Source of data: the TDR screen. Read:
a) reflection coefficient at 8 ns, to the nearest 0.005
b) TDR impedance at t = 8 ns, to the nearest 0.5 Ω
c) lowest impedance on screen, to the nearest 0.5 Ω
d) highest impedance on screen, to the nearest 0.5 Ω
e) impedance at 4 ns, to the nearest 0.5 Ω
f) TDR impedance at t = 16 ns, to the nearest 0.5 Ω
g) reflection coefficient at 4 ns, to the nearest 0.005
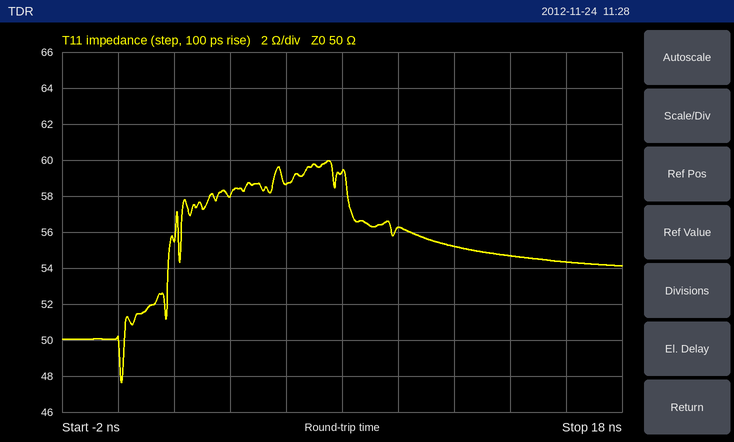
+0.085
59.5 Ω
47.5 Ω
60.0 Ω
58.0 Ω
54.5 Ω
+0.075
